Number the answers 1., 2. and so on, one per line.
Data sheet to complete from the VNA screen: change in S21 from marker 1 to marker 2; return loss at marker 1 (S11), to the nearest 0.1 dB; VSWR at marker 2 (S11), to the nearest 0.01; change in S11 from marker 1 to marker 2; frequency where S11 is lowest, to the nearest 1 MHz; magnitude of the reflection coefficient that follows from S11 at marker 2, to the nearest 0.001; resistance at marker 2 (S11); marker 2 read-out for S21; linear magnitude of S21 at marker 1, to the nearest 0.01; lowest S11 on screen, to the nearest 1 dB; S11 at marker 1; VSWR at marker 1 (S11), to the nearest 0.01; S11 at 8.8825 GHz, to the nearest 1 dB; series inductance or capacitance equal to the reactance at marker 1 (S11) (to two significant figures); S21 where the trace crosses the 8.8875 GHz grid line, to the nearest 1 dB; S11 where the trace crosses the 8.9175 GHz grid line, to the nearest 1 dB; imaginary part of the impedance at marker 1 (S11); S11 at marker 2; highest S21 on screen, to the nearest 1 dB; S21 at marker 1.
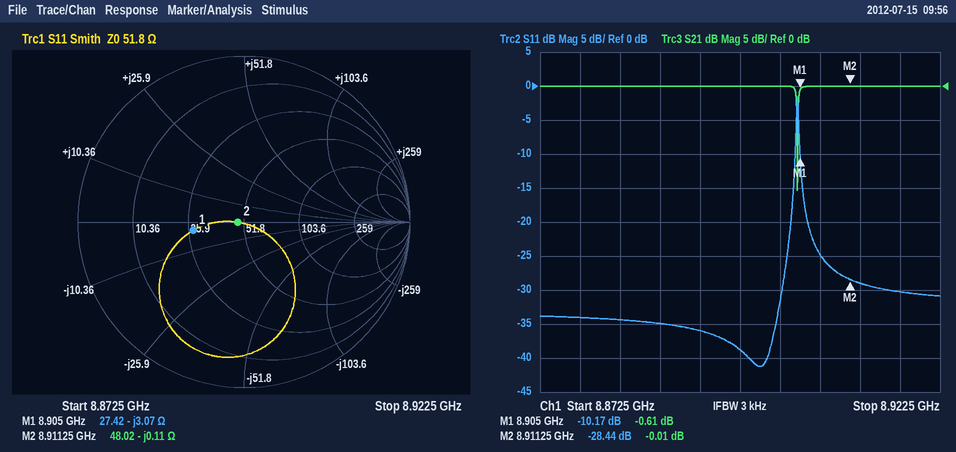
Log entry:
1. 0.60 dB
2. 10.2 dB
3. 1.08
4. -18.27 dB
5. 8.900 GHz
6. 0.038
7. 48.02 Ω
8. -0.01 dB
9. 0.93
10. -41 dB
11. -10.17 dB
12. 1.90
13. -34 dB
14. 5.8 pF
15. 0 dB
16. -30 dB
17. -3.07 Ω
18. -28.44 dB
19. 0 dB
20. -0.61 dB
